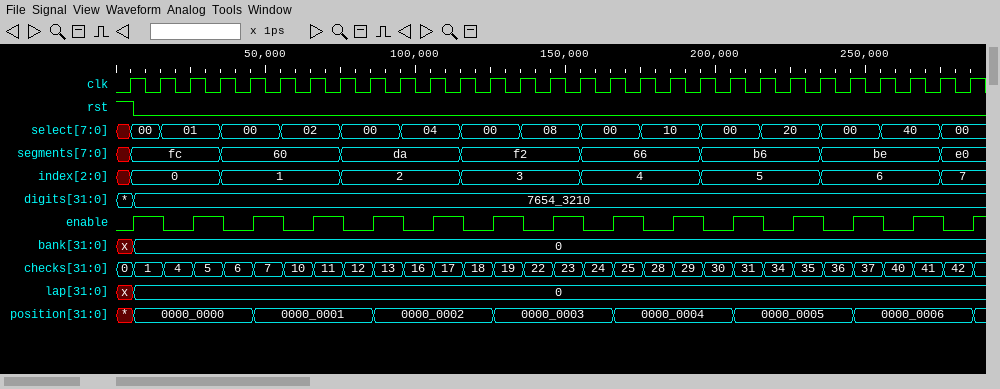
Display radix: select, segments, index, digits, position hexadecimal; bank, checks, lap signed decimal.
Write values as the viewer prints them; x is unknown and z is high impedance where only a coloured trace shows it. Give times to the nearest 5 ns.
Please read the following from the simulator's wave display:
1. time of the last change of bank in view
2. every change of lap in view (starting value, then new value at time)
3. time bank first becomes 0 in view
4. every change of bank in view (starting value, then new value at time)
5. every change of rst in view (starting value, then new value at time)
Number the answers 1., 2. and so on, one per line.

1. 5 ns
2. x, 0 at 5 ns
3. 5 ns
4. x, 0 at 5 ns
5. 1, 0 at 5 ns
